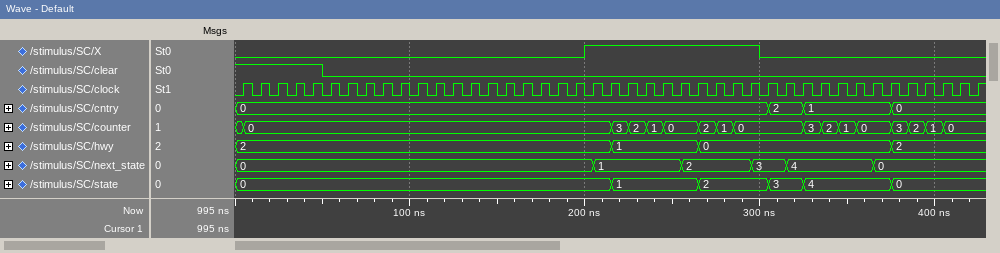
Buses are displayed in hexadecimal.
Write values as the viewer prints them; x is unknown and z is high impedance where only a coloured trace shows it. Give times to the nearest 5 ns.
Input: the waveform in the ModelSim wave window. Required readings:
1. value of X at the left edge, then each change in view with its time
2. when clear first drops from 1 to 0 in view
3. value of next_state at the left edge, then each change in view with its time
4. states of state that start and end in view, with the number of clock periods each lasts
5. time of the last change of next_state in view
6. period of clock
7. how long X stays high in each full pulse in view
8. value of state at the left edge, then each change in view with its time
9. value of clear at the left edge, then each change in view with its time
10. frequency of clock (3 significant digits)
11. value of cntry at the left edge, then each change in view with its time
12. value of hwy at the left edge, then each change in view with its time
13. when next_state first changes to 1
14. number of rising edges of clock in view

0, 1 at 200 ns, 0 at 300 ns
50 ns
0, 1 at 205 ns, 2 at 255 ns, 3 at 295 ns, 4 at 315 ns, 0 at 365 ns
1: 5, 2: 4, 3: 2, 4: 5
365 ns
10 ns
100 ns
0, 1 at 215 ns, 2 at 265 ns, 3 at 305 ns, 4 at 325 ns, 0 at 375 ns
1, 0 at 50 ns
100 MHz
0, 2 at 305 ns, 1 at 325 ns, 0 at 375 ns
2, 1 at 215 ns, 0 at 265 ns, 2 at 375 ns
205 ns
43
